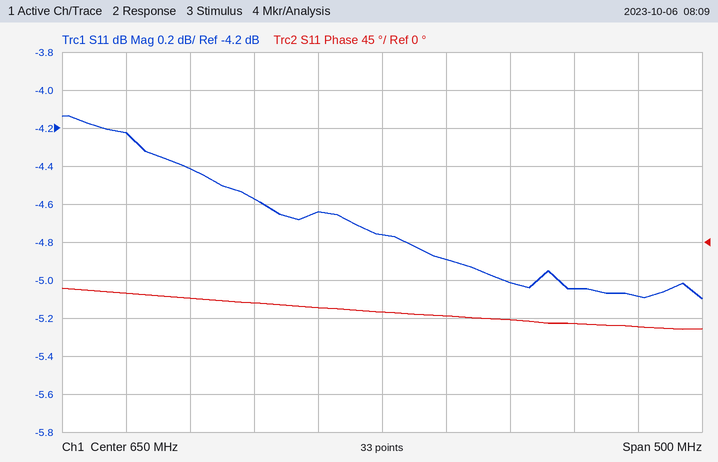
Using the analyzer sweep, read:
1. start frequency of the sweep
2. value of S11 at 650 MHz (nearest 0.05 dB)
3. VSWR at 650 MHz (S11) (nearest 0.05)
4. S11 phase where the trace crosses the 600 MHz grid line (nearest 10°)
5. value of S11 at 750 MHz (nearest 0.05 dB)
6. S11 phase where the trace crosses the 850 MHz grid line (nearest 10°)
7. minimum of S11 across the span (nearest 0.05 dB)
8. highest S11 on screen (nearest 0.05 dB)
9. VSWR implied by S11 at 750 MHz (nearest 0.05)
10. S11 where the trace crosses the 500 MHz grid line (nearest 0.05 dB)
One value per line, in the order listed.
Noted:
400 MHz
-4.75 dB
3.75
-80°
-5.00 dB
-100°
-5.10 dB
-4.15 dB
3.55
-4.40 dB
